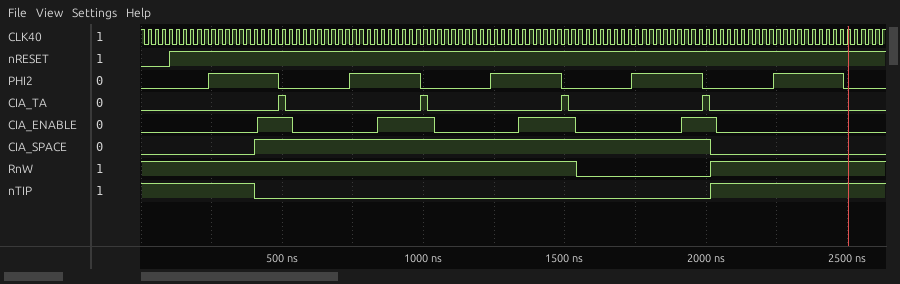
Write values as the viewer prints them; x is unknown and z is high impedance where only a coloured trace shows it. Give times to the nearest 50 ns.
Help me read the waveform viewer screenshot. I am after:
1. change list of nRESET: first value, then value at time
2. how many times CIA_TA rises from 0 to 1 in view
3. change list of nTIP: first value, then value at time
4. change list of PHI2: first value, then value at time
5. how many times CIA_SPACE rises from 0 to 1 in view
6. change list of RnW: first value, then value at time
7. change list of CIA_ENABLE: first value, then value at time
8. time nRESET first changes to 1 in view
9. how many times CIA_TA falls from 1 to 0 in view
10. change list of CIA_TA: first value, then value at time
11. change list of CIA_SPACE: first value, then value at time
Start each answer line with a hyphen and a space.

- 0, 1 at 100 ns
- 4
- 1, 0 at 400 ns, 1 at 2000 ns
- 0, 1 at 250 ns, 0 at 500 ns, 1 at 750 ns, 0 at 1000 ns, 1 at 1250 ns, 0 at 1500 ns, 1 at 1750 ns, 0 at 2000 ns, 1 at 2250 ns, 0 at 2500 ns
- 1
- 1, 0 at 1550 ns, 1 at 2000 ns
- 0, 1 at 400 ns, 0 at 550 ns, 1 at 850 ns, 0 at 1050 ns, 1 at 1350 ns, 0 at 1550 ns, 1 at 1900 ns, 0 at 2050 ns
- 100 ns
- 4
- 0, 1 at 500 ns, 0 at 500 ns, 1 at 1000 ns, 0 at 1000 ns, 1 at 1500 ns, 0 at 1500 ns, 1 at 2000 ns, 0 at 2000 ns
- 0, 1 at 400 ns, 0 at 2000 ns
